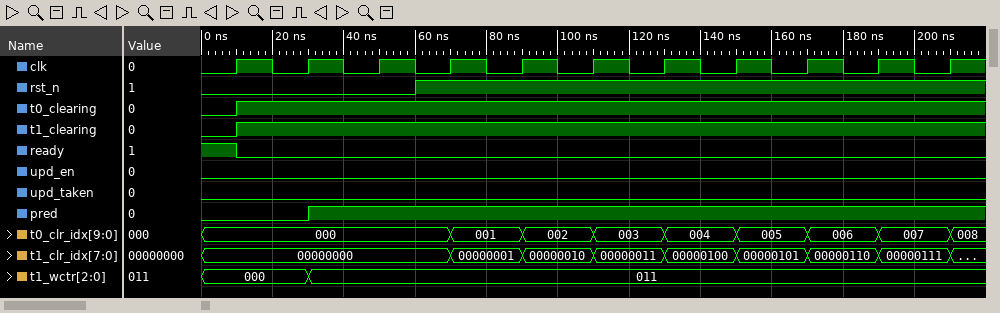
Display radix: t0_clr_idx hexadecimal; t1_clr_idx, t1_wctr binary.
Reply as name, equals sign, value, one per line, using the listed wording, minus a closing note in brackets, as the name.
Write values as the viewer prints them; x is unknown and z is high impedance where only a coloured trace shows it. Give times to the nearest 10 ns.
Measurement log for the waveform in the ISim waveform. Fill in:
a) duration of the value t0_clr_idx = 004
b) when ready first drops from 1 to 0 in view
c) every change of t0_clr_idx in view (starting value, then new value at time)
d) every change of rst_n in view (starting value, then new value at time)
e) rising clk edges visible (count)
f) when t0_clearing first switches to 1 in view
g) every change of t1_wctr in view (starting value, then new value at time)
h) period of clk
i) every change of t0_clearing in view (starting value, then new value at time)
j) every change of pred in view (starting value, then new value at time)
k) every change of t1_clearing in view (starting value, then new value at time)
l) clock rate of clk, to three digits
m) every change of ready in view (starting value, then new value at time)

duration of the value t0_clr_idx = 004 = 20 ns
when ready first drops from 1 to 0 in view = 10 ns
every change of t0_clr_idx in view = 000, 001 at 70 ns, 002 at 90 ns, 003 at 110 ns, 004 at 130 ns, 005 at 150 ns, 006 at 170 ns, 007 at 190 ns, 008 at 210 ns
every change of rst_n in view = 0, 1 at 60 ns
rising clk edges visible = 11
when t0_clearing first switches to 1 in view = 10 ns
every change of t1_wctr in view = 000, 011 at 30 ns
period of clk = 20 ns
every change of t0_clearing in view = 0, 1 at 10 ns
every change of pred in view = 0, 1 at 30 ns
every change of t1_clearing in view = 0, 1 at 10 ns
clock rate of clk, to three digits = 50.0 MHz
every change of ready in view = 1, 0 at 10 ns
